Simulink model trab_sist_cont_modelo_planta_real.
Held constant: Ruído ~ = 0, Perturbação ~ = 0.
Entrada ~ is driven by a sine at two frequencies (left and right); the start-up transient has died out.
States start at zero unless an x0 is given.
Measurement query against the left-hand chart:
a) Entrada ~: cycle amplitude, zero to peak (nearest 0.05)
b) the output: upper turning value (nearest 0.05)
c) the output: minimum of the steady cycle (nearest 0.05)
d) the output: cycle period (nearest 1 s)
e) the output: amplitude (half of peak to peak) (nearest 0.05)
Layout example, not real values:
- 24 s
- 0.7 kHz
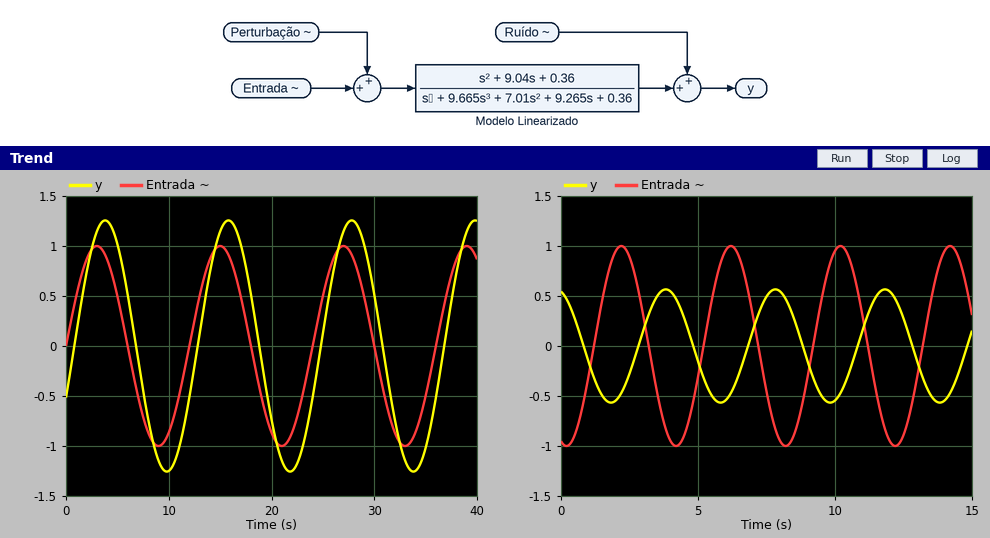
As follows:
- 1.00
- 1.25
- -1.25
- 12 s
- 1.25
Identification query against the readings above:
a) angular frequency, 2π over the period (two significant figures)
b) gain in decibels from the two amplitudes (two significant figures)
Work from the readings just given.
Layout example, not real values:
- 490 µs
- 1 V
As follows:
- 0.52 rad/s
- 1.9 dB
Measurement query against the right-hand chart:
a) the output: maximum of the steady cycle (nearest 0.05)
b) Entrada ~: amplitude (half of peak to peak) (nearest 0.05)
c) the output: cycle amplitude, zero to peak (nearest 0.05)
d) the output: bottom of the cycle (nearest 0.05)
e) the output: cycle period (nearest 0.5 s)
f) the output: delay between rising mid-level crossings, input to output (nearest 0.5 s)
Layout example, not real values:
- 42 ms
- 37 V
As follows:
- 0.55
- 1.00
- 0.55
- -0.55
- 4.0 s
- 1.5 s
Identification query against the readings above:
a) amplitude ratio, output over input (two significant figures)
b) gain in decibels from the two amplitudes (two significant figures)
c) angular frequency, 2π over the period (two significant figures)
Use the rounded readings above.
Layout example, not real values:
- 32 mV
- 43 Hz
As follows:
- 0.55
- -5.2 dB
- 1.6 rad/s
